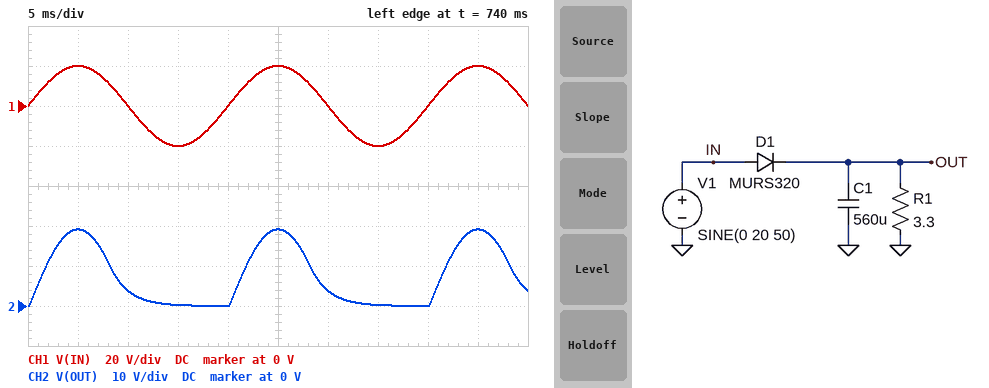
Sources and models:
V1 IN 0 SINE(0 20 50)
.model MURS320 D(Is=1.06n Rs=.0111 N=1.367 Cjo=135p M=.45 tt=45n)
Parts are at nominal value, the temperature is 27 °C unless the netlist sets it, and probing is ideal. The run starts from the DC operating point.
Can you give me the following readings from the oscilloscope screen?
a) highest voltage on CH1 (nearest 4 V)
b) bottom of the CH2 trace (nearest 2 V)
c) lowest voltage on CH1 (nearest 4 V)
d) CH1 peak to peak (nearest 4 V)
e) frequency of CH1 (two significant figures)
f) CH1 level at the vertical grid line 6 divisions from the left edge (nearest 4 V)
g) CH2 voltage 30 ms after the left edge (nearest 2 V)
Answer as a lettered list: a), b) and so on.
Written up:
a) 20 V
b) 0 V
c) -20 V
d) 40 V
e) 50 Hz
f) 0 V
g) 4 V
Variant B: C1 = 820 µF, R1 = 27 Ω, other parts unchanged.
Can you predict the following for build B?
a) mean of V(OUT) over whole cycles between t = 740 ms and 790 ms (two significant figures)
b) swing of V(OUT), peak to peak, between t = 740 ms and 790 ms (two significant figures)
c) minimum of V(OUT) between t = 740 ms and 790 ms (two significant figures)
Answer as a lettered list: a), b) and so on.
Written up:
a) 14 V
b) 10 V
c) 9.2 V
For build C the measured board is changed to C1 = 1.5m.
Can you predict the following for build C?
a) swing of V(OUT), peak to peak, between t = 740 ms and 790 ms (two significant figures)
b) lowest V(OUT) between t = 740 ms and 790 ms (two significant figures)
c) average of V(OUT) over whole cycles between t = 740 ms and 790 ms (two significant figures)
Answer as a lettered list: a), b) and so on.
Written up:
a) 18 V
b) 1.1 V
c) 8.3 V
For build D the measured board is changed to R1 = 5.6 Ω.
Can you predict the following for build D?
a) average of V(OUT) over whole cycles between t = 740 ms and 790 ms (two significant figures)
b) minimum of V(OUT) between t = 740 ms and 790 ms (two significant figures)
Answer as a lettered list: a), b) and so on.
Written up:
a) 7.2 V
b) 240 mV
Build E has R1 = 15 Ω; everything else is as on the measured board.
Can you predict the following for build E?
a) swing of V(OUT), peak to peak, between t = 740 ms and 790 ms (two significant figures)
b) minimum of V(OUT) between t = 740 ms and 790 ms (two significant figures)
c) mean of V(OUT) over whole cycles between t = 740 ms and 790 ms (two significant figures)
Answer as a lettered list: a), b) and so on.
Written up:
a) 16 V
b) 3.2 V
c) 10 V
